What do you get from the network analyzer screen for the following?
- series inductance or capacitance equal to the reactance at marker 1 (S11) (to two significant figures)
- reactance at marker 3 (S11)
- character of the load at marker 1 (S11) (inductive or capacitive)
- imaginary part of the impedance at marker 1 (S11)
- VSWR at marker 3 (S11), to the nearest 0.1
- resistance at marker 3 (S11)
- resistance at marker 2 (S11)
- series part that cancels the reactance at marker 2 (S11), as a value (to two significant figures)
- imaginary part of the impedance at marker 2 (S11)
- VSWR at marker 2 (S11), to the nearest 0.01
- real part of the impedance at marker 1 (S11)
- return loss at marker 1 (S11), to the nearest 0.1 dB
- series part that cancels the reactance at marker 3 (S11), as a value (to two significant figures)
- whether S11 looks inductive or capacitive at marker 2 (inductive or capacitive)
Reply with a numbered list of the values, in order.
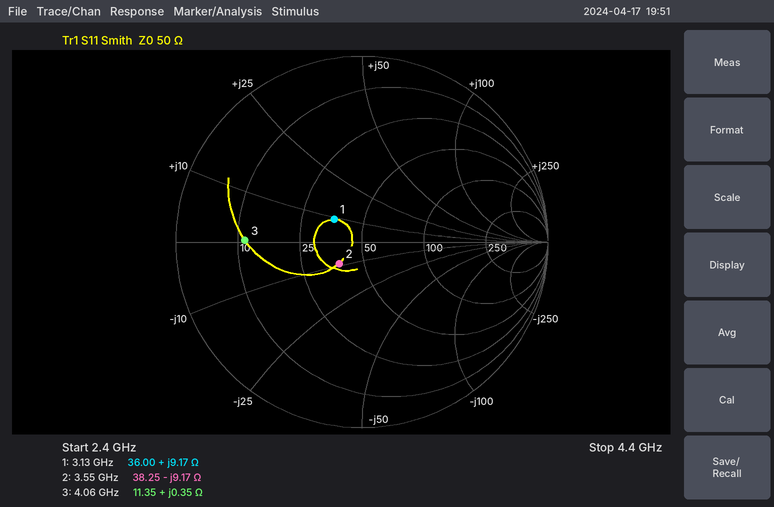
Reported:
1. 470 pH
2. +0.35 Ω
3. inductive
4. +9.17 Ω
5. 4.4
6. 11.35 Ω
7. 38.25 Ω
8. 410 pH
9. -9.17 Ω
10. 1.40
11. 36.00 Ω
12. 14.3 dB
13. 110 pF
14. capacitive
